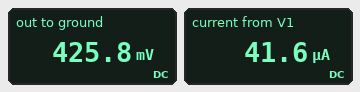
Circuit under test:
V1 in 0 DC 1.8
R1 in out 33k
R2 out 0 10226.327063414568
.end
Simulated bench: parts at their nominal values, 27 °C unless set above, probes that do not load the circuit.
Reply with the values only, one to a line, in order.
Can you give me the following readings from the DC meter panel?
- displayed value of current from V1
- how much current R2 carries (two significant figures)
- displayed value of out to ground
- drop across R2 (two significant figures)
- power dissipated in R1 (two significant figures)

41.6 µA
42 µA
425.8 mV
430 mV
57 µW
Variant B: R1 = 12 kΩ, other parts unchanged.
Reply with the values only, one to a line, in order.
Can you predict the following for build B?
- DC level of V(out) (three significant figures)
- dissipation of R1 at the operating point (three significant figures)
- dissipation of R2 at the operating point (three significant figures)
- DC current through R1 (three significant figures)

828 mV
78.7 µW
67.1 µW
81.0 µA
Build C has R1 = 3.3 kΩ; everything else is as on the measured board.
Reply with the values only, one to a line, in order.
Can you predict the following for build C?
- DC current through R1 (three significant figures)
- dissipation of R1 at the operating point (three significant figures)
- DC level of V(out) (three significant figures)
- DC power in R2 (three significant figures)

133 µA
58.4 µW
1.36 V
181 µW
